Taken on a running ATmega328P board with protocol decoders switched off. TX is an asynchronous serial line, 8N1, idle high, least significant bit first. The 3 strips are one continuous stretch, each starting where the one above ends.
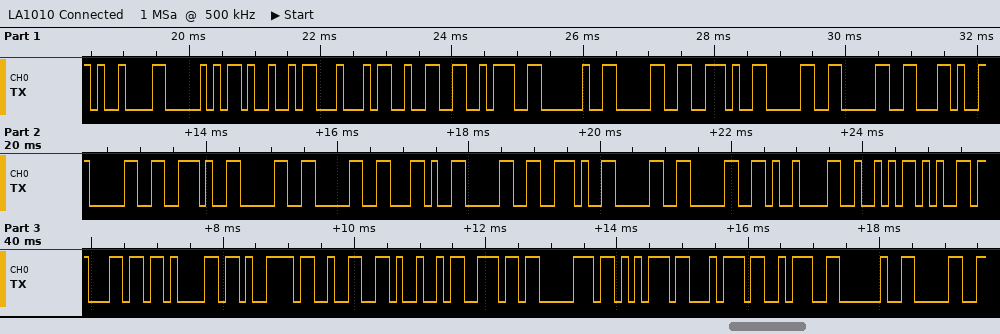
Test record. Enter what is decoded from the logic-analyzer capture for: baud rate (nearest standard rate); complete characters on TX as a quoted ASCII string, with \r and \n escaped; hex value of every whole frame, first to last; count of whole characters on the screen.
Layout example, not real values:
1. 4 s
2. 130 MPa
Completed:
1. 9600 baud
2. "\tPID2: 0.00,0.00,0.00\tRelay2Input: 0"
3. 09 50 49 44 32 3A 20 30 2E 30 30 2C 30 2E 30 30 2C 30 2E 30 30 09 52 65 6C 61 79 32 49 6E 70 75 74 3A 20 30
4. 36
